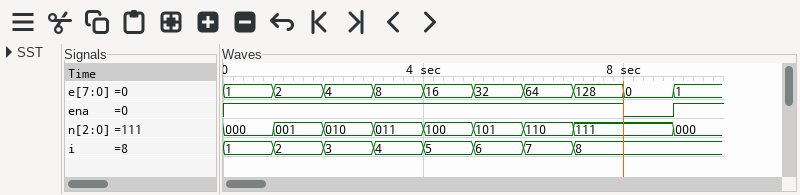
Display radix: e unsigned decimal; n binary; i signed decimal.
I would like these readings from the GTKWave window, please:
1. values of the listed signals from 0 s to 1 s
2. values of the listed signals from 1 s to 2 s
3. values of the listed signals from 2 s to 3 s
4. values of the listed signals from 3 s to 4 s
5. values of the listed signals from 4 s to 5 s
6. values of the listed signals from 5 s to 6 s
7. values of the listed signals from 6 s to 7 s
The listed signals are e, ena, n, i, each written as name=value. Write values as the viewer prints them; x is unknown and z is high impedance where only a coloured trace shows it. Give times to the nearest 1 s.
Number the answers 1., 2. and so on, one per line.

1. e=1, ena=1, n=000, i=1
2. e=2, ena=1, n=001, i=2
3. e=4, ena=1, n=010, i=3
4. e=8, ena=1, n=011, i=4
5. e=16, ena=1, n=100, i=5
6. e=32, ena=1, n=101, i=6
7. e=64, ena=1, n=110, i=7
